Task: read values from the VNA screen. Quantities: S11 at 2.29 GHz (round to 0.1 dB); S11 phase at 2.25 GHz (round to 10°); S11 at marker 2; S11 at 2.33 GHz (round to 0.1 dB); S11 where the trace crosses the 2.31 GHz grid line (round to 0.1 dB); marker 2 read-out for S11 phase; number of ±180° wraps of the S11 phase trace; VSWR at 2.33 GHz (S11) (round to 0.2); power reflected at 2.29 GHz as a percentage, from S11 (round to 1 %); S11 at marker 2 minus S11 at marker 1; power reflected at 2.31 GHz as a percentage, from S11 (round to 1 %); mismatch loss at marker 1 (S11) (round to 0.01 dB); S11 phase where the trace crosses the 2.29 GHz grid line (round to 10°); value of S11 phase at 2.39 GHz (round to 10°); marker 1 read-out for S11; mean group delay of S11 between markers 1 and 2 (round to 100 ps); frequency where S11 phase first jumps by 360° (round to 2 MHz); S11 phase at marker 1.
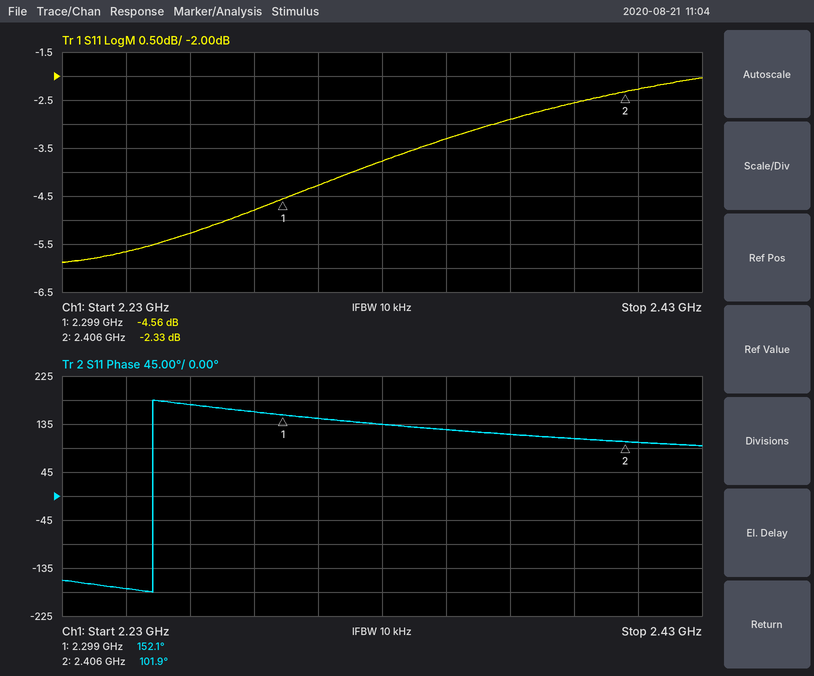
-4.8 dB
-170°
-2.33 dB
-3.8 dB
-4.3 dB
101.9°
1
4.6
33 %
2.23 dB
37 %
1.87 dB
160°
110°
-4.56 dB
1.3 ns
2.258 GHz
152.1°
